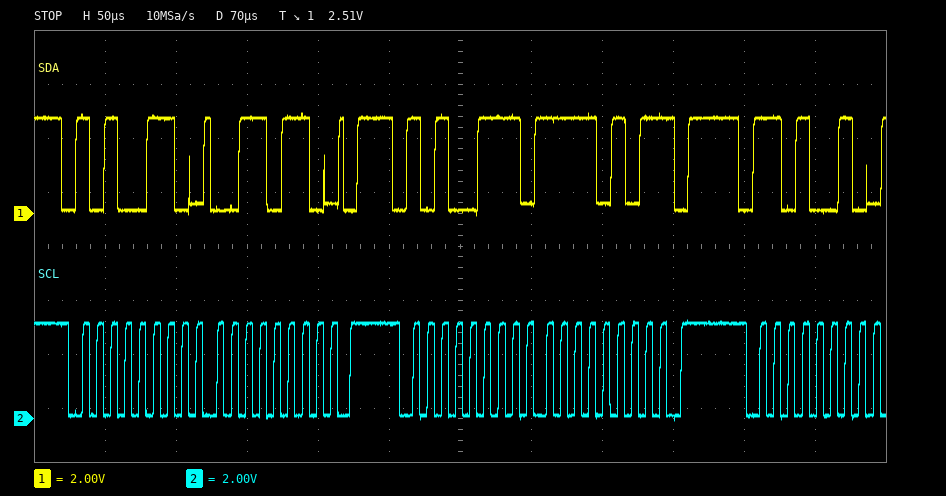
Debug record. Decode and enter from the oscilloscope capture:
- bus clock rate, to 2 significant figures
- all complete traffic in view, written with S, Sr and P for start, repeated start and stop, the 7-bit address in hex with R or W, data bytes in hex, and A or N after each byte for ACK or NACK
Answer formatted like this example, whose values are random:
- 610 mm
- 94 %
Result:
- 100 kHz
- S 53W A 36 A P S 53R A F5 N P S 69W A
